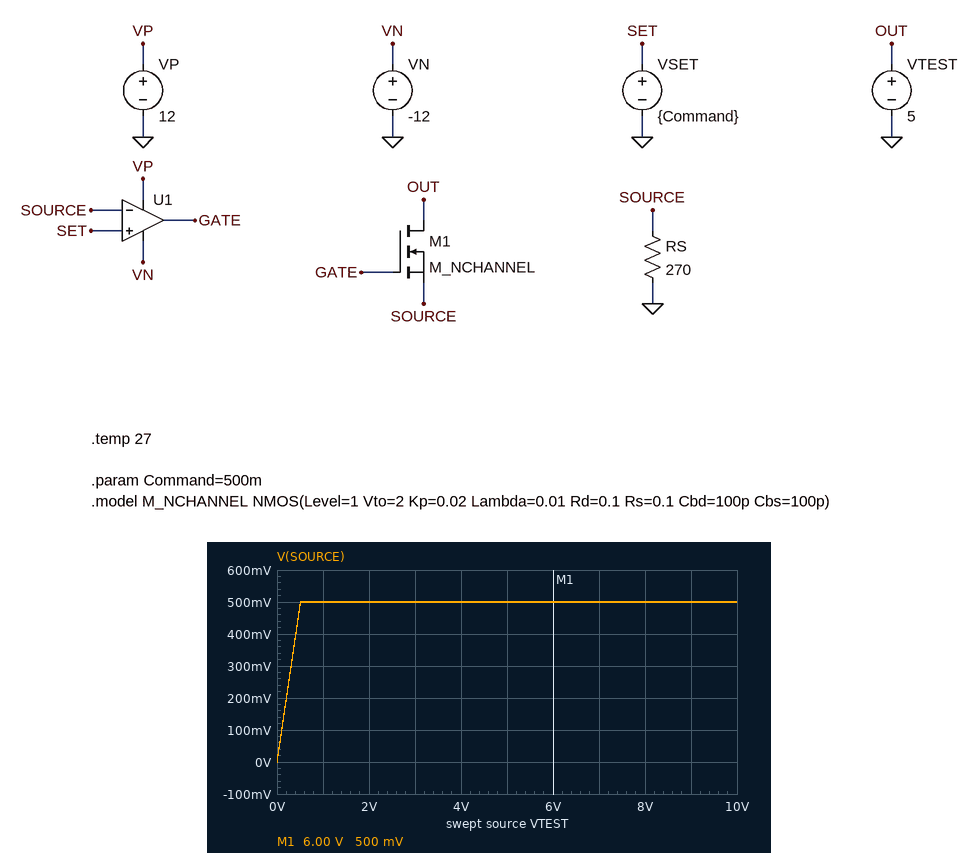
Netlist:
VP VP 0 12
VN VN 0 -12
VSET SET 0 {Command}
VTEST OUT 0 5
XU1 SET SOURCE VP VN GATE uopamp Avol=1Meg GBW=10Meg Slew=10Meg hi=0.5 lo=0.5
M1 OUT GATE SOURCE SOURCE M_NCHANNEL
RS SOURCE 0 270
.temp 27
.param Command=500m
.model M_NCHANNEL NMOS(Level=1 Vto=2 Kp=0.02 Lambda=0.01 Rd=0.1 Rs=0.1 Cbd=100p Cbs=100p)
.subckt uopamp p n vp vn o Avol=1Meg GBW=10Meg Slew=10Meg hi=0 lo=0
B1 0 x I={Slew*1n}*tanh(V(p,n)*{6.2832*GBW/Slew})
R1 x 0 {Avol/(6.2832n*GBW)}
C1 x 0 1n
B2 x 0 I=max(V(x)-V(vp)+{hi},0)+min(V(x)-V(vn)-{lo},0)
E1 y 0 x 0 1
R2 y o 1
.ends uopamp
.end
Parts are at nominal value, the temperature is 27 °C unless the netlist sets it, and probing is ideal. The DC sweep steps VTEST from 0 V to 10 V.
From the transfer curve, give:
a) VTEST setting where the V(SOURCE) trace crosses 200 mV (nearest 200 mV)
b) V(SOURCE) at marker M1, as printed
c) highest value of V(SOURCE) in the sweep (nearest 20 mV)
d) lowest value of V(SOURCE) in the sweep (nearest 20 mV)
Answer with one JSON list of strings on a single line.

["200 mV", "500 mV", "500 mV", "0 V"]
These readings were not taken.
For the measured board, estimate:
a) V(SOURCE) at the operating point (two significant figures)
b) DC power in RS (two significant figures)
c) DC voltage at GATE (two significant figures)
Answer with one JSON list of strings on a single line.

["500 mV", "930 µW", "2.9 V"]
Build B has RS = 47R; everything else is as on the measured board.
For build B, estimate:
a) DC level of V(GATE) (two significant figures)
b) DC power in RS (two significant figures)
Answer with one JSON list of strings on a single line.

["3.5 V", "5.3 mW"]
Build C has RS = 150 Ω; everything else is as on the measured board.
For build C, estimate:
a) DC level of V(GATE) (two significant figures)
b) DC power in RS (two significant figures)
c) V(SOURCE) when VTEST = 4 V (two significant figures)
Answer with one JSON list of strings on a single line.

["3.1 V", "1.7 mW", "500 mV"]
